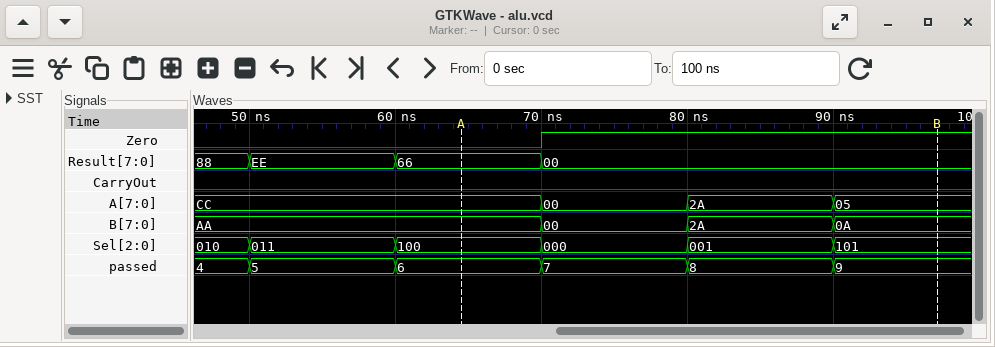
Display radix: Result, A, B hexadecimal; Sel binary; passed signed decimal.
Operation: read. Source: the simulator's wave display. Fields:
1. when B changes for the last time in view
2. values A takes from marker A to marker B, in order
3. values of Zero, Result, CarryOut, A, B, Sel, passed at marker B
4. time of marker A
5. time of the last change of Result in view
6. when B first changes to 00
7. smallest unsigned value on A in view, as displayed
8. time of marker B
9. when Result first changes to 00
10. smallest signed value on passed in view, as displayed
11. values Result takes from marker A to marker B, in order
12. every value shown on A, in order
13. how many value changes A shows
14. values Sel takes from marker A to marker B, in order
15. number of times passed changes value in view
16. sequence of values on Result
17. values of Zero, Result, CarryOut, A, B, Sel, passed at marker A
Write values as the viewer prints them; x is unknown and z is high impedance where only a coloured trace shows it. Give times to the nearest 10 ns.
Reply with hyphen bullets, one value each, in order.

- 90 ns
- CC, 00, 2A, 05
- Zero=1, Result=00, CarryOut=0, A=05, B=0A, Sel=101, passed=9
- 60 ns
- 70 ns
- 70 ns
- 00
- 100 ns
- 70 ns
- 4
- 66, 00
- CC, 00, 2A, 05
- 3
- 100, 000, 001, 101
- 5
- 88, EE, 66, 00
- Zero=0, Result=66, CarryOut=0, A=CC, B=AA, Sel=100, passed=6
